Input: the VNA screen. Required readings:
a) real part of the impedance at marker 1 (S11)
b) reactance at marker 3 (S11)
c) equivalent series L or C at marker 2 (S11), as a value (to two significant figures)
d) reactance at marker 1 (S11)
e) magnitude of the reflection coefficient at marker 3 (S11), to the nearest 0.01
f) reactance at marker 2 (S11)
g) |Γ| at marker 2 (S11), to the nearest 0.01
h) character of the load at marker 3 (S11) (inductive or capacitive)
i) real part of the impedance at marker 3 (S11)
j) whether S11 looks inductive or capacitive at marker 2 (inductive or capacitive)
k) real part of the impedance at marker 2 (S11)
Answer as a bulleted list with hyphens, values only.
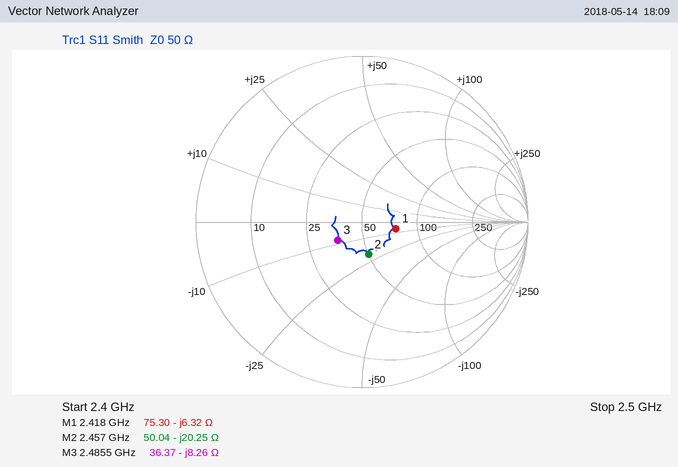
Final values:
- 75.30 Ω
- -8.26 Ω
- 3.2 pF
- -6.32 Ω
- 0.18
- -20.25 Ω
- 0.20
- capacitive
- 36.37 Ω
- capacitive
- 50.04 Ω
